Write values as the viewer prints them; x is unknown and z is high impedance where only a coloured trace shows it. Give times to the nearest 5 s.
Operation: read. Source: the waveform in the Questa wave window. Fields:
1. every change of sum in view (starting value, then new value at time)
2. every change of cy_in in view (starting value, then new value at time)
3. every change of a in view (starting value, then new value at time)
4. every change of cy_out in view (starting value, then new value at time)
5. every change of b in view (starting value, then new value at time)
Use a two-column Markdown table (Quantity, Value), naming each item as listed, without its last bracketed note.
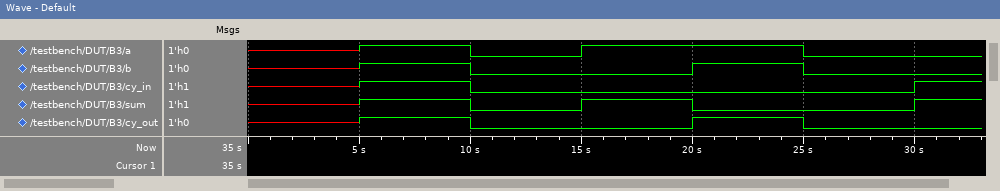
| Quantity | Value |
|---|---|
| every change of sum in view | x, 1 at 5 s, 0 at 10 s, 1 at 15 s, 0 at 20 s, 1 at 30 s |
| every change of cy_in in view | x, 1 at 5 s, 0 at 10 s, 1 at 30 s |
| every change of a in view | x, 1 at 5 s, 0 at 10 s, 1 at 15 s, 0 at 25 s |
| every change of cy_out in view | x, 1 at 5 s, 0 at 10 s, 1 at 20 s, 0 at 25 s |
| every change of b in view | x, 1 at 5 s, 0 at 10 s, 1 at 20 s, 0 at 25 s |
